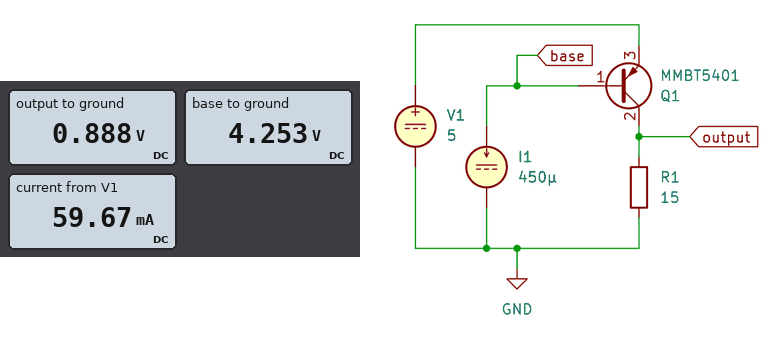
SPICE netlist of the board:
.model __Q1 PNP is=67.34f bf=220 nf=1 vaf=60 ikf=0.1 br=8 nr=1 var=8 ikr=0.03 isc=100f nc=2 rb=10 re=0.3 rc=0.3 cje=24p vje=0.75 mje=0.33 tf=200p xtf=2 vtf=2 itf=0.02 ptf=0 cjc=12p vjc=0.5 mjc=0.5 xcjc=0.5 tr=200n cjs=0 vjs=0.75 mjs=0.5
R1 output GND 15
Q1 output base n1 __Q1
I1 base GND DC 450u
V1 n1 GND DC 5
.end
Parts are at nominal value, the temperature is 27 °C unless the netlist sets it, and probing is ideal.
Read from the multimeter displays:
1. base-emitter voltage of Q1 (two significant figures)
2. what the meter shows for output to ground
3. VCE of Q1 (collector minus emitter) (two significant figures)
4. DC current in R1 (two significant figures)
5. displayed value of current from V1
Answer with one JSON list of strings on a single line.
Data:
["-750 mV", "0.888 V", "-4.1 V", "59 mA", "59.67 mA"]
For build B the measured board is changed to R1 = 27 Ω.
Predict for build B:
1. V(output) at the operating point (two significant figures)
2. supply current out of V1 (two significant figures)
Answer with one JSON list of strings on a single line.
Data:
["1.6 V", "59 mA"]
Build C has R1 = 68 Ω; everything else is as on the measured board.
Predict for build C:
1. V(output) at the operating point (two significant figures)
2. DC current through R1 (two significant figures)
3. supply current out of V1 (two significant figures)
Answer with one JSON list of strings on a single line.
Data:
["3.8 V", "56 mA", "57 mA"]
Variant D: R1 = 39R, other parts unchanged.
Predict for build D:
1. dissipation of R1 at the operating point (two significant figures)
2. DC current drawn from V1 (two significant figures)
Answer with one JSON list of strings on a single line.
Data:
["130 mW", "58 mA"]
